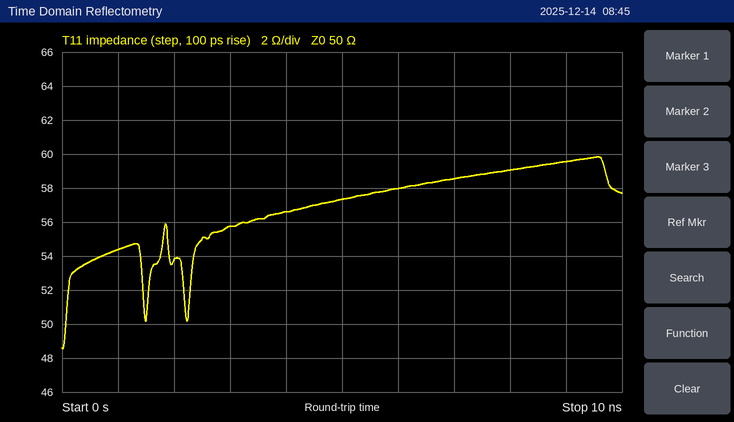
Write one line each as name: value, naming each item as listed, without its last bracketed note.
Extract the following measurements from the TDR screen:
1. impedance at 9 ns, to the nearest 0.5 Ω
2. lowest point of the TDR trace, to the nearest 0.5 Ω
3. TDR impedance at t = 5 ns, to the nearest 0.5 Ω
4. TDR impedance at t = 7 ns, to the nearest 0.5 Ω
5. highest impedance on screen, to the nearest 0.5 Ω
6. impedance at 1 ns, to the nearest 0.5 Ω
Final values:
impedance at 9 ns, to the nearest 0.5 Ω: 59.5 Ω
lowest point of the TDR trace, to the nearest 0.5 Ω: 48.5 Ω
TDR impedance at t = 5 ns, to the nearest 0.5 Ω: 57.5 Ω
TDR impedance at t = 7 ns, to the nearest 0.5 Ω: 58.5 Ω
highest impedance on screen, to the nearest 0.5 Ω: 60.0 Ω
impedance at 1 ns, to the nearest 0.5 Ω: 54.5 Ω
